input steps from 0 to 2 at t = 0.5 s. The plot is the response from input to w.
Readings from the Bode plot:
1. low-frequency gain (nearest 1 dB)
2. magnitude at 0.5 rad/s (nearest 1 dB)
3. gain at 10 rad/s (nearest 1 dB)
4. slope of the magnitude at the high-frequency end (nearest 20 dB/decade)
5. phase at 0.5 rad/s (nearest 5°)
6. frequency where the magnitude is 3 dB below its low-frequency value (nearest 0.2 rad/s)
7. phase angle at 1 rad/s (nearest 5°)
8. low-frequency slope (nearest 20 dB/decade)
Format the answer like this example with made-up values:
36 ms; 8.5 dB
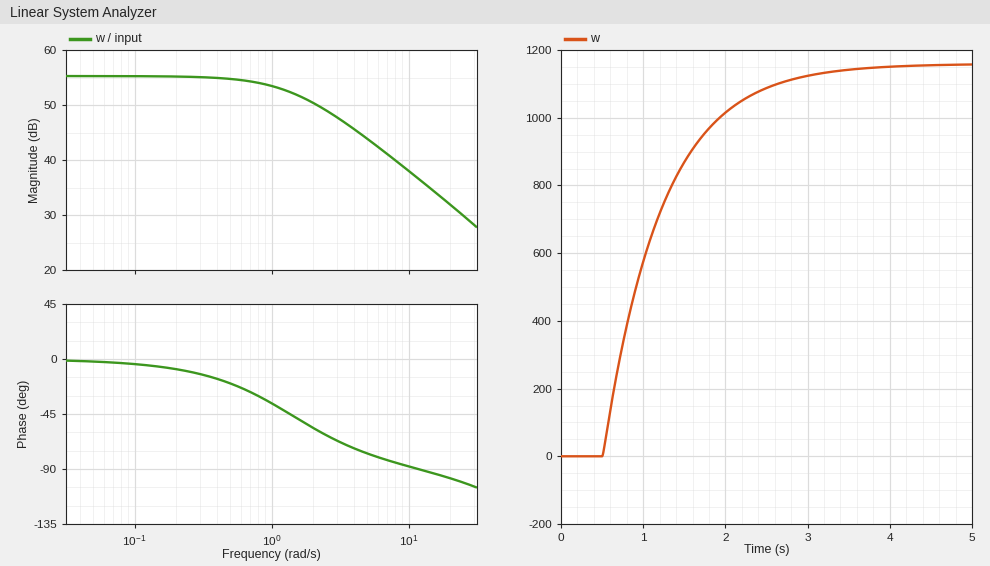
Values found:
55 dB; 55 dB; 38 dB; -20 dB/decade; -20°; 1.4 rad/s; -35°; 0 dB/decade
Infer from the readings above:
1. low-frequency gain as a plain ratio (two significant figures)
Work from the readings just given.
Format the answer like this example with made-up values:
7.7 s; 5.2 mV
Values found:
560
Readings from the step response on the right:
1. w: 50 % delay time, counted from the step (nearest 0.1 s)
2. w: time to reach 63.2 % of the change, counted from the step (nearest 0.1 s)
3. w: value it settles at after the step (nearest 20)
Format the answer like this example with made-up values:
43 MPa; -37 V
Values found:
0.5 s; 0.7 s; 1160
